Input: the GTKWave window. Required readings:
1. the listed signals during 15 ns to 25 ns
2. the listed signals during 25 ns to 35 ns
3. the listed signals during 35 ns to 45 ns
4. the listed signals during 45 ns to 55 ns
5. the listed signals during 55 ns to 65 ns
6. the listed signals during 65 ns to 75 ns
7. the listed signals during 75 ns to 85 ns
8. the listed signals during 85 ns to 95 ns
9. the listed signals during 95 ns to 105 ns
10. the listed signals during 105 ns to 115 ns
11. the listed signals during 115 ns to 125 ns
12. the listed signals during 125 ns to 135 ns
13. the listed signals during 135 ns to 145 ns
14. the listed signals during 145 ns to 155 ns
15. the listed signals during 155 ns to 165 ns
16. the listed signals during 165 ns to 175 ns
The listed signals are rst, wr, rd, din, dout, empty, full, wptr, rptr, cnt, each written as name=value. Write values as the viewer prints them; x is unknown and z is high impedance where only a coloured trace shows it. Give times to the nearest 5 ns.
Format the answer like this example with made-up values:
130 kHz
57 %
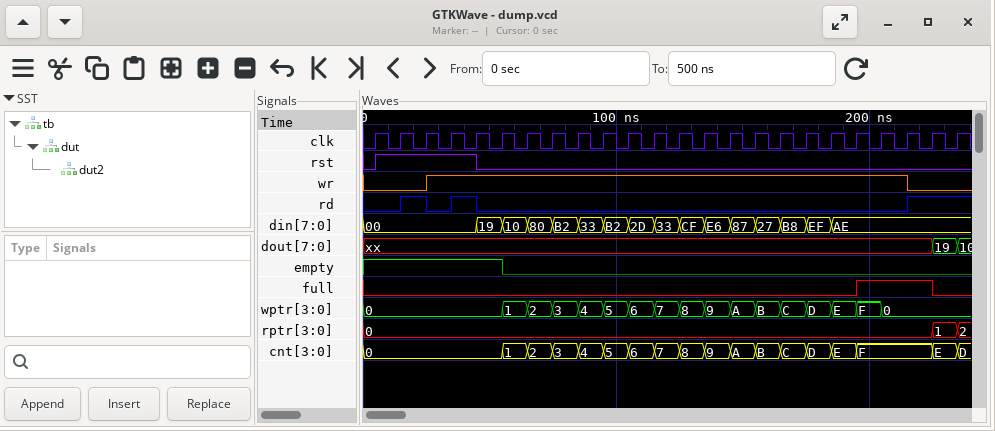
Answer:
rst=1, wr=0, rd=1, din=00, dout=xx, empty=1, full=0, wptr=0, rptr=0, cnt=0
rst=1, wr=1, rd=0, din=00, dout=xx, empty=1, full=0, wptr=0, rptr=0, cnt=0
rst=1, wr=1, rd=1, din=00, dout=xx, empty=1, full=0, wptr=0, rptr=0, cnt=0
rst=0, wr=1, rd=0, din=19, dout=xx, empty=1, full=0, wptr=0, rptr=0, cnt=0
rst=0, wr=1, rd=0, din=10, dout=xx, empty=0, full=0, wptr=1, rptr=0, cnt=1
rst=0, wr=1, rd=0, din=80, dout=xx, empty=0, full=0, wptr=2, rptr=0, cnt=2
rst=0, wr=1, rd=0, din=B2, dout=xx, empty=0, full=0, wptr=3, rptr=0, cnt=3
rst=0, wr=1, rd=0, din=33, dout=xx, empty=0, full=0, wptr=4, rptr=0, cnt=4
rst=0, wr=1, rd=0, din=B2, dout=xx, empty=0, full=0, wptr=5, rptr=0, cnt=5
rst=0, wr=1, rd=0, din=2D, dout=xx, empty=0, full=0, wptr=6, rptr=0, cnt=6
rst=0, wr=1, rd=0, din=33, dout=xx, empty=0, full=0, wptr=7, rptr=0, cnt=7
rst=0, wr=1, rd=0, din=CF, dout=xx, empty=0, full=0, wptr=8, rptr=0, cnt=8
rst=0, wr=1, rd=0, din=E6, dout=xx, empty=0, full=0, wptr=9, rptr=0, cnt=9
rst=0, wr=1, rd=0, din=87, dout=xx, empty=0, full=0, wptr=A, rptr=0, cnt=A
rst=0, wr=1, rd=0, din=27, dout=xx, empty=0, full=0, wptr=B, rptr=0, cnt=B
rst=0, wr=1, rd=0, din=B8, dout=xx, empty=0, full=0, wptr=C, rptr=0, cnt=C
